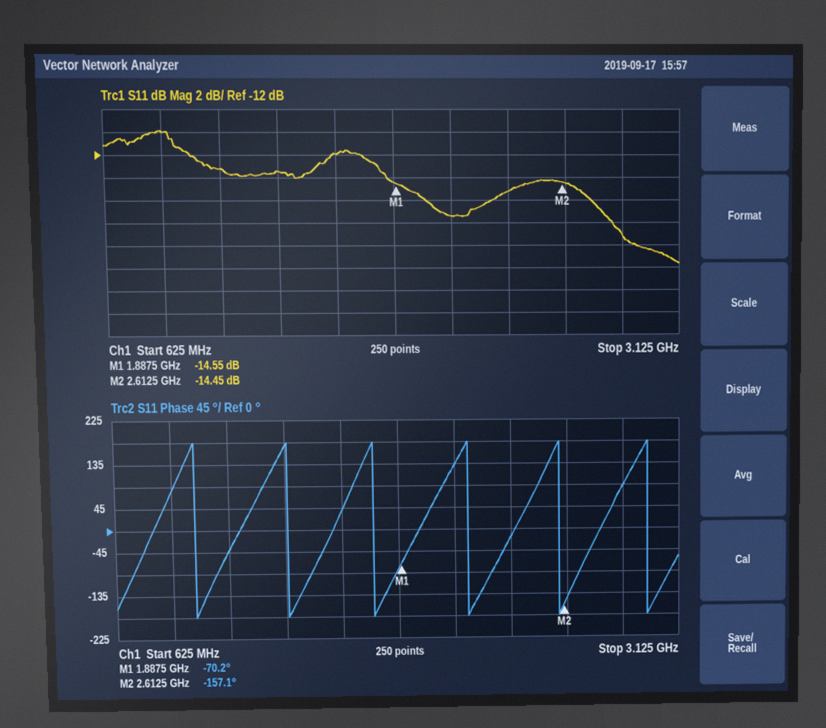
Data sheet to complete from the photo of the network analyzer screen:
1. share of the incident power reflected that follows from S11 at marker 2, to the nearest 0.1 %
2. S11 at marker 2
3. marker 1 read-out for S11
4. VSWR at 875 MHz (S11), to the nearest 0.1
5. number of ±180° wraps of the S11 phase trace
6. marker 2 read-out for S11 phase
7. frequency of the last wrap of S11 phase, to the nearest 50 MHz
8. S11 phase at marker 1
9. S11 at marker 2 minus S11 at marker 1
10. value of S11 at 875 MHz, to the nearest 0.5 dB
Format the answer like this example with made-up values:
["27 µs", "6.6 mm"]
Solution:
["3.6 %", "-14.45 dB", "-14.55 dB", "1.9", "6", "-157.1°", "3.00 GHz", "-70.2°", "0.10 dB", "-10.0 dB"]
